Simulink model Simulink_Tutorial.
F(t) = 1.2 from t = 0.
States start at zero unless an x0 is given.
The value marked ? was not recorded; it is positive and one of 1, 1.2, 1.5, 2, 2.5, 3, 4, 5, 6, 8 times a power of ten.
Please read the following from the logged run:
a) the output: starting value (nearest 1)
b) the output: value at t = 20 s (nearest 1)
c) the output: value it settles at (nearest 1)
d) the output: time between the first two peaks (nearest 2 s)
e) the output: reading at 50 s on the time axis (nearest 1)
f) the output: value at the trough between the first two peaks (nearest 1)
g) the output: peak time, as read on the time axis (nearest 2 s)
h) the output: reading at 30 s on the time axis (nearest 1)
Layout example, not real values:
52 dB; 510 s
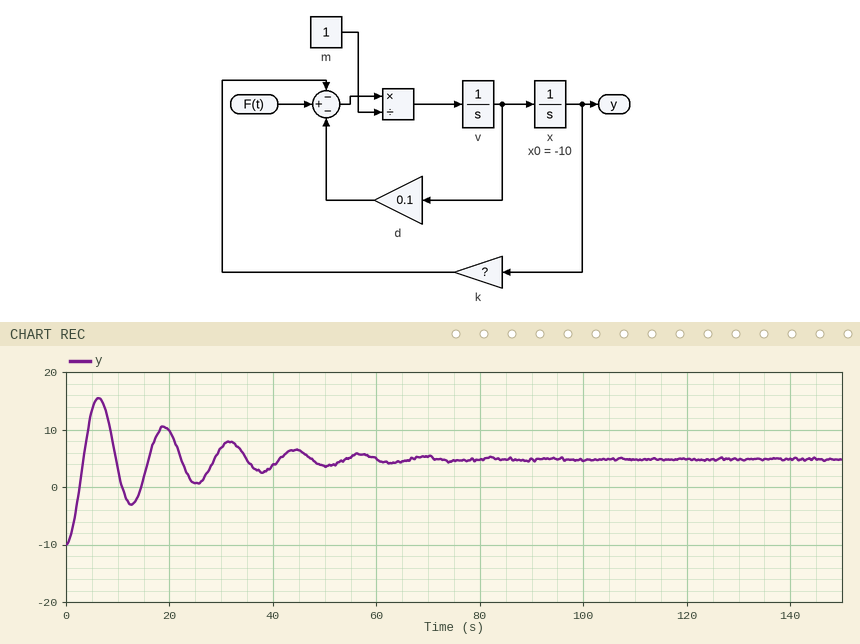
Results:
-10; 10; 5; 12 s; 4; -3; 6 s; 7
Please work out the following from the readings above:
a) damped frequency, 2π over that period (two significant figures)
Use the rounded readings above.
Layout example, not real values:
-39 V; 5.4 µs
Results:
0.52 rad/s
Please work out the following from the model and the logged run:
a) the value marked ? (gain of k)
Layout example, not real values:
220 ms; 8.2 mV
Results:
0.25
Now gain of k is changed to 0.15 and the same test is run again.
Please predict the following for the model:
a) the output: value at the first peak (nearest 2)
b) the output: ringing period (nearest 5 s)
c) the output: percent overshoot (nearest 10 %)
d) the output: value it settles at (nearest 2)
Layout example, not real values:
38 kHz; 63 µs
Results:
20; 15 s; 70 %; 8
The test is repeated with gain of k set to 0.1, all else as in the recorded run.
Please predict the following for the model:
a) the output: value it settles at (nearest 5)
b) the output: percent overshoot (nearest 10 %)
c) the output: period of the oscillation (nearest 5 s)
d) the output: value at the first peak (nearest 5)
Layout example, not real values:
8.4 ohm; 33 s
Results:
10; 60 %; 20 s; 25
